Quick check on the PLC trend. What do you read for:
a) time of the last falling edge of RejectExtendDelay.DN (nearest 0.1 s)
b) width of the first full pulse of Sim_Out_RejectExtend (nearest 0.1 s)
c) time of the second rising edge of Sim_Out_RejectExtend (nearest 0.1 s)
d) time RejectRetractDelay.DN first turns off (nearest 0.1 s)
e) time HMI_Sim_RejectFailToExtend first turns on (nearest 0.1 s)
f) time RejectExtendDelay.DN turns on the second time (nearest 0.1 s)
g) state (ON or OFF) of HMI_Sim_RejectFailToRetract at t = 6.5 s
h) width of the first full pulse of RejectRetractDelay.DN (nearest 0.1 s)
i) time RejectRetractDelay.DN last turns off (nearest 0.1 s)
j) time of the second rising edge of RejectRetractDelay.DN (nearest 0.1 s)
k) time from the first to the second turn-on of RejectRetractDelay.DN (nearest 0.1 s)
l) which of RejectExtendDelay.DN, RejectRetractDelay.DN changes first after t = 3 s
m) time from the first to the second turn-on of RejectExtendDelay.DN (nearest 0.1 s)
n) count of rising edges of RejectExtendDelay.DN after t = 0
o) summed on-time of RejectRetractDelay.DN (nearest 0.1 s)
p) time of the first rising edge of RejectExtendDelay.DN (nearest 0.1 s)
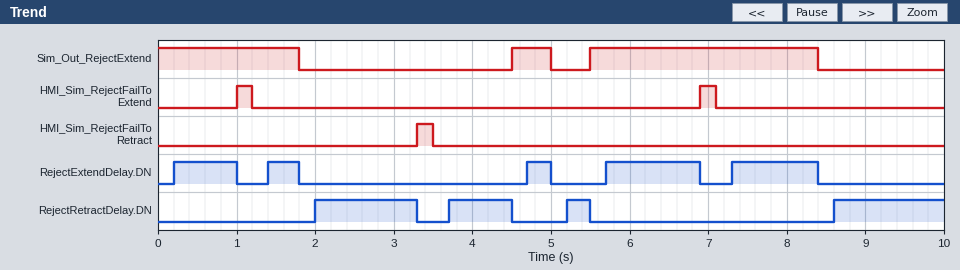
8.4 s
0.5 s
5.5 s
3.3 s
1.0 s
1.4 s
OFF
1.3 s
5.5 s
3.7 s
1.7 s
RejectRetractDelay.DN
1.2 s
5
3.8 s
0.2 s
